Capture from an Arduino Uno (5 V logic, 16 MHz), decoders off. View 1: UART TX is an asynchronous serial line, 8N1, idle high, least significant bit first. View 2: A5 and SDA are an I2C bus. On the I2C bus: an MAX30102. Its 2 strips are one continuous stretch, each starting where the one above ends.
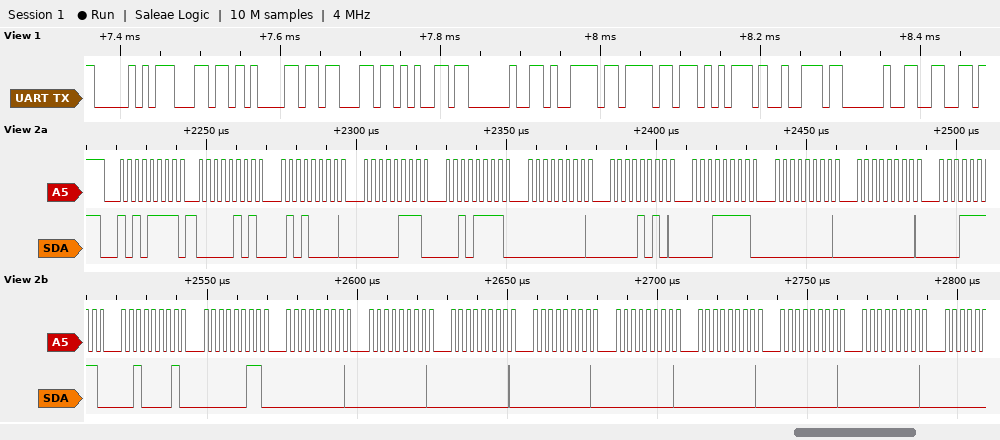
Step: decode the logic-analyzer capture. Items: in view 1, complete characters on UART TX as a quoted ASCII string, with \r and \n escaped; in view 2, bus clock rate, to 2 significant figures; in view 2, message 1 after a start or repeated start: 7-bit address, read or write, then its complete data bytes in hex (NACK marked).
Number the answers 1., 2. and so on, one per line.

1. "Place your f"
2. 400 kHz
3. 0x57 read: 05 50 07 2F 00 0A 1F 00 00 1F 21 03 00 00 00 00 00 00 00 00
